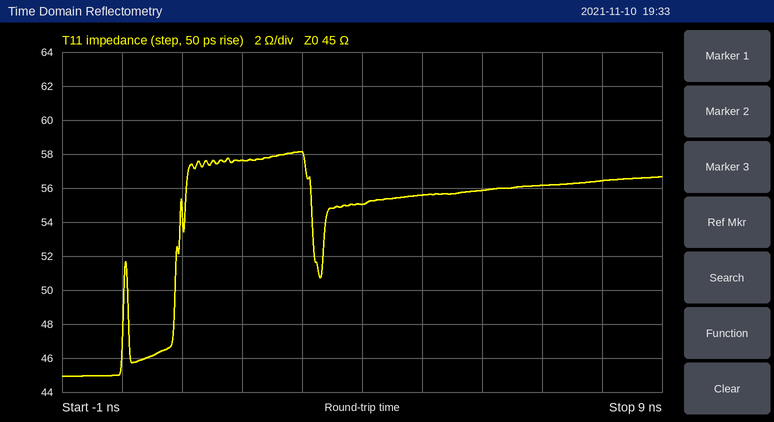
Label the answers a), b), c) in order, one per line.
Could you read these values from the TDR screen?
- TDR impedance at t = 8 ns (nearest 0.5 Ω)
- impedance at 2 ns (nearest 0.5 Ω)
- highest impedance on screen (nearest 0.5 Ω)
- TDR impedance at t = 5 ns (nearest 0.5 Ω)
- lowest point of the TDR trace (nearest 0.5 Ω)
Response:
a) 56.5 Ω
b) 57.5 Ω
c) 58.0 Ω
d) 55.5 Ω
e) 45.0 Ω
